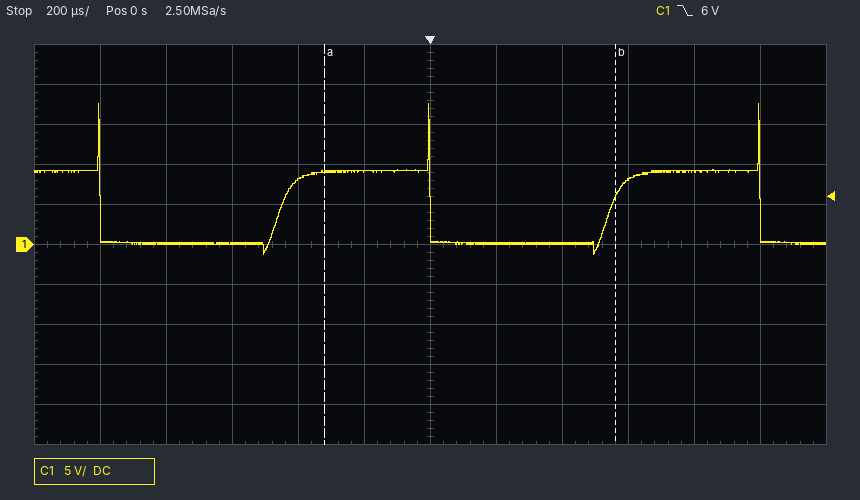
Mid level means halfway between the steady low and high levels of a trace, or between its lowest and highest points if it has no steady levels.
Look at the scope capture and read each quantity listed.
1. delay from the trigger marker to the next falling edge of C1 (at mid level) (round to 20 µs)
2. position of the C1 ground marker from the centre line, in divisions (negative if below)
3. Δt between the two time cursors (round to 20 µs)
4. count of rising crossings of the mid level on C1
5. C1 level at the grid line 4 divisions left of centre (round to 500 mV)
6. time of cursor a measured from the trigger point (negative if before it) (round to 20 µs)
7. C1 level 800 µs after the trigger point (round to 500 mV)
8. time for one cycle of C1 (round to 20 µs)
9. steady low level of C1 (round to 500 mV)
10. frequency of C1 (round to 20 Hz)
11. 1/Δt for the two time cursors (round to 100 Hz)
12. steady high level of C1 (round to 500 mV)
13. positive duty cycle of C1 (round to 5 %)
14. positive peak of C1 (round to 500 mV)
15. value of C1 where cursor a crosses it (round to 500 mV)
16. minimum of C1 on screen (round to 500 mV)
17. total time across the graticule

1.00 ms
0.0 div
880 µs
2
0.0 V
-320 µs
9.0 V
1.00 ms
0.0 V
1.00 kHz
1.1 kHz
9.0 V
45 %
17.5 V
9.0 V
-1.0 V
2.4 ms
